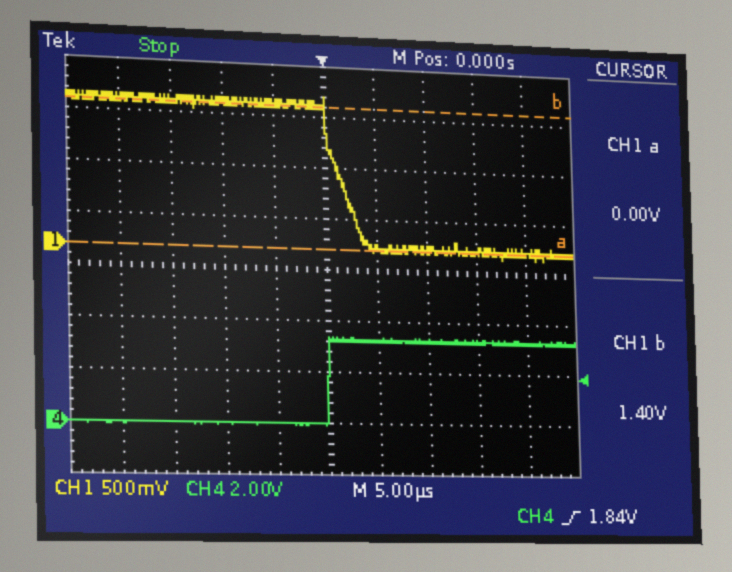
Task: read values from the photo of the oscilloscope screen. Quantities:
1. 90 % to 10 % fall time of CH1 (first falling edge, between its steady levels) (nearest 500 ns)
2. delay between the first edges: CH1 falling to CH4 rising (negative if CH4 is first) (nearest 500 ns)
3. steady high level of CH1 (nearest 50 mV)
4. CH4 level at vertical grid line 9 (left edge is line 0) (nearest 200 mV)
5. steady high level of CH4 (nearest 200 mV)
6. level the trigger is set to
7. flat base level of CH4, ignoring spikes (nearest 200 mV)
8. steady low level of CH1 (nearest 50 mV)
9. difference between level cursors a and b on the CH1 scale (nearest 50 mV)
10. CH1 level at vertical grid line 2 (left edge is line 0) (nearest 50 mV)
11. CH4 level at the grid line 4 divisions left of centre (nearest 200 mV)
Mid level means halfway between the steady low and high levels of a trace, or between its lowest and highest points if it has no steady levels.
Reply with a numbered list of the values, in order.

1. 3.5 µs
2. -1.5 µs
3. 1.40 V
4. 3.2 V
5. 3.2 V
6. 1.84 V
7. 0.0 V
8. 0 mV
9. 1.40 V
10. 1.40 V
11. 0.0 V
